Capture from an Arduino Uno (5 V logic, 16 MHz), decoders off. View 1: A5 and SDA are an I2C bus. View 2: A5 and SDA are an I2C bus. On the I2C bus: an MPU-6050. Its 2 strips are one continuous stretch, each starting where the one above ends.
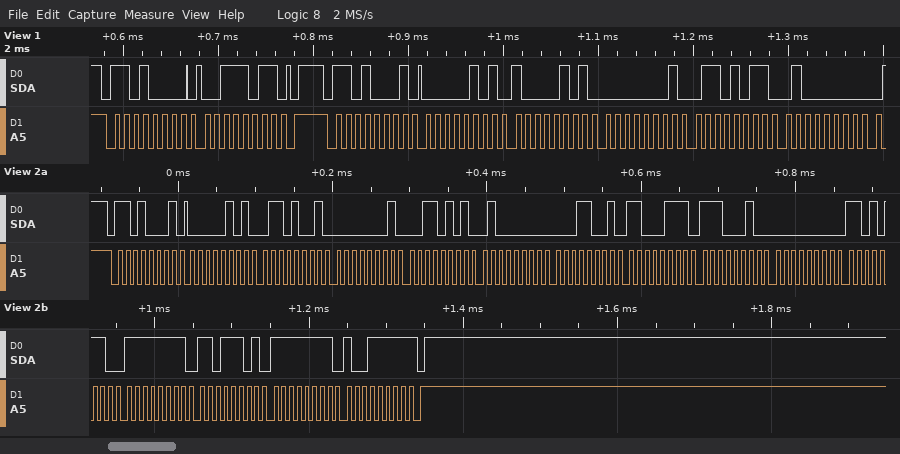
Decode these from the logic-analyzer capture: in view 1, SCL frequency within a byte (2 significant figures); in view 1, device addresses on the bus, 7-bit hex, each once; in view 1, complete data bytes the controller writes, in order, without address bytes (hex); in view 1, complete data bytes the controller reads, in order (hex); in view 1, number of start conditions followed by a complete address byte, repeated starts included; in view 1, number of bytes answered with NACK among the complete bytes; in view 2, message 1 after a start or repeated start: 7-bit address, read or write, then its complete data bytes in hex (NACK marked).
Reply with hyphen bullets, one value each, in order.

- 100 kHz
- 0x68
- 3B
- 05 85 01 6B 40
- 2
- 0
- 0x68 read: 05 69 01 35 40 19 C7 E2 00 D6 FF DD FF 9F NACK
